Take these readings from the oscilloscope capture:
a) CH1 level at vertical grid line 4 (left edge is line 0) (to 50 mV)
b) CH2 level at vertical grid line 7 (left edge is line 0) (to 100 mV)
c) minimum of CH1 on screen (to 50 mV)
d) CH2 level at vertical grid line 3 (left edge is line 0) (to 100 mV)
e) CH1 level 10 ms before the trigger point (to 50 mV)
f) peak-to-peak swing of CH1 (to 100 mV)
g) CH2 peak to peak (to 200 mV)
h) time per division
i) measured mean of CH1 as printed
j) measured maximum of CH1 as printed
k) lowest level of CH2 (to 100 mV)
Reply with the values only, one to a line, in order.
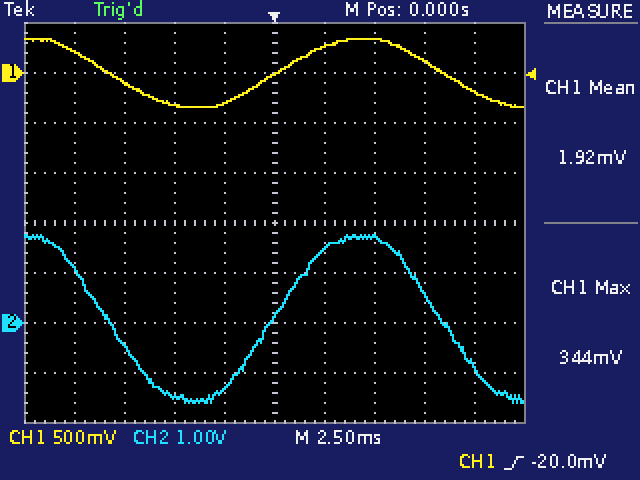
-300 mV
1.7 V
-350 mV
-1.5 V
200 mV
700 mV
3.4 V
2.5 ms
1.92 mV
344 mV
-1.6 V
